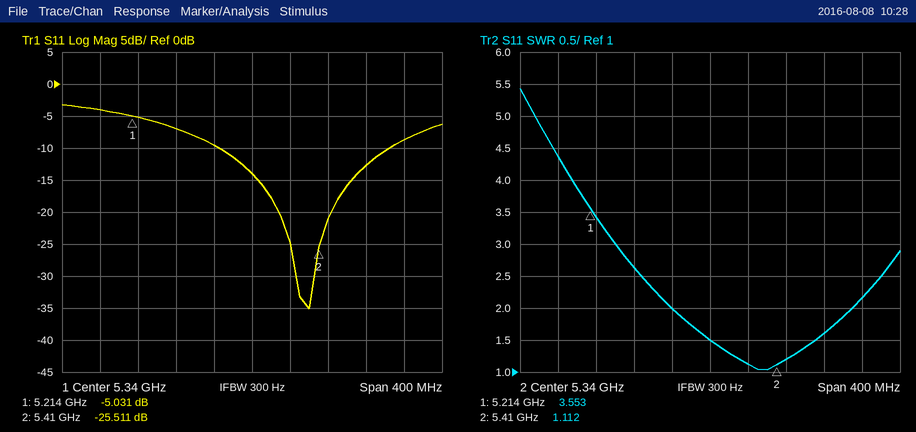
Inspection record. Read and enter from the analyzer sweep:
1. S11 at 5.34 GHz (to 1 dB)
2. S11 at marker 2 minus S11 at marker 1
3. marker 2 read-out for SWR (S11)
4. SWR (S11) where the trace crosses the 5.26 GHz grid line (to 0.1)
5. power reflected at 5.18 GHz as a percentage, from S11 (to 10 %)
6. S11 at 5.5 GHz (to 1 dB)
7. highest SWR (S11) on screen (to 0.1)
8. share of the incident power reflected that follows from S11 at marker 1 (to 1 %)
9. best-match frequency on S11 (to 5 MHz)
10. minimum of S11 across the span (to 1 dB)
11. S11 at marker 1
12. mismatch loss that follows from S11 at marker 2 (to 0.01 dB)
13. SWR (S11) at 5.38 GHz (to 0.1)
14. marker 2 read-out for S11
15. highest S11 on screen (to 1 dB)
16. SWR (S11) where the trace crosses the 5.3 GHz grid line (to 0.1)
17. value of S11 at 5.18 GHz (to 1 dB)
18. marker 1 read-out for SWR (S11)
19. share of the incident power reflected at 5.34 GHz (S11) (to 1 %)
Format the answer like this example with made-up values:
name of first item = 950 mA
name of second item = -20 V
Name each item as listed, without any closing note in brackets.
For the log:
S11 at 5.34 GHz = -14 dB
S11 at marker 2 minus S11 at marker 1 = -20.480 dB
marker 2 read-out for SWR = 1.112
SWR (S11) where the trace crosses the 5.26 GHz grid line = 2.6
power reflected at 5.18 GHz as a percentage, from S11 = 40 %
S11 at 5.5 GHz = -9 dB
highest SWR (S11) on screen = 5.4
share of the incident power reflected that follows from S11 at marker 1 = 31 %
best-match frequency on S11 = 5.400 GHz
minimum of S11 across the span = -35 dB
S11 at marker 1 = -5.031 dB
mismatch loss that follows from S11 at marker 2 = 0.01 dB
SWR (S11) at 5.38 GHz = 1.1
marker 2 read-out for S11 = -25.511 dB
highest S11 on screen = -3 dB
SWR (S11) where the trace crosses the 5.3 GHz grid line = 2.0
value of S11 at 5.18 GHz = -4 dB
marker 1 read-out for SWR = 3.553
share of the incident power reflected at 5.34 GHz (S11) = 4 %
